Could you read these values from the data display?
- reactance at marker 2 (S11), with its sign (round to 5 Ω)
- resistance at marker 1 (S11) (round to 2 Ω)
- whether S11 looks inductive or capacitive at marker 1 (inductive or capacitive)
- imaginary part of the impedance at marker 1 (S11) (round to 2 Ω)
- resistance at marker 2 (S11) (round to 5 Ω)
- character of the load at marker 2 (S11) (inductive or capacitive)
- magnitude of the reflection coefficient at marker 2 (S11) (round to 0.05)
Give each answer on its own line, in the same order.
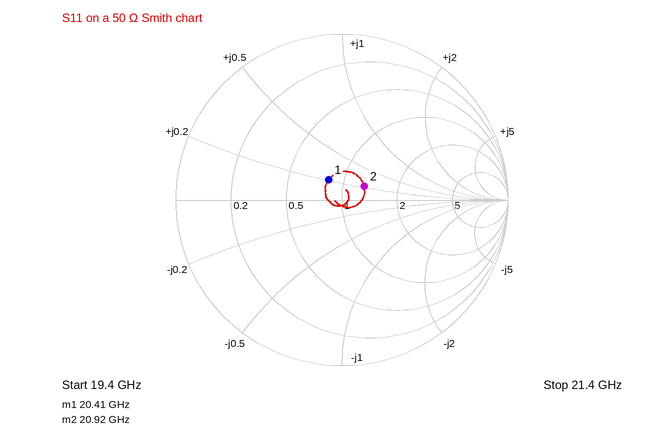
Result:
+10 Ω
42 Ω
inductive
+10 Ω
65 Ω
inductive
0.15
